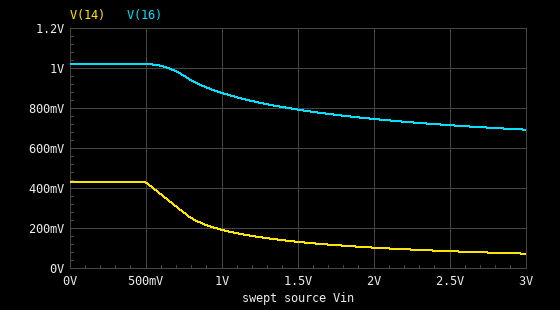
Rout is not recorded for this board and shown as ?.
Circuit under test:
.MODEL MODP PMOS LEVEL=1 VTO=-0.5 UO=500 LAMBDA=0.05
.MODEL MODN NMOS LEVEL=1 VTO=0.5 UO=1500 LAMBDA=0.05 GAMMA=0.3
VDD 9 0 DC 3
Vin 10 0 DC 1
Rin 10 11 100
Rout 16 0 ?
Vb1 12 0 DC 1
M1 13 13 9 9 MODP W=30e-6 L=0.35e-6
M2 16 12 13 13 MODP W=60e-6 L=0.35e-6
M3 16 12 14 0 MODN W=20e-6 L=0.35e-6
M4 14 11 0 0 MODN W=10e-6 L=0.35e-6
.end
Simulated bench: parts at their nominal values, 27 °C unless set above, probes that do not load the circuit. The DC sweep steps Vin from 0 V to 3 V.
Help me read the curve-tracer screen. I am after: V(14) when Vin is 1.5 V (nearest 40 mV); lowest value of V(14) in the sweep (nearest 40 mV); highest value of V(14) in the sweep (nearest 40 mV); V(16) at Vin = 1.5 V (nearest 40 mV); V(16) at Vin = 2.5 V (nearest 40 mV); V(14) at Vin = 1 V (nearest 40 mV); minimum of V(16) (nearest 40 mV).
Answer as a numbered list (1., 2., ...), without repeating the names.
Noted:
1. 120 mV
2. 80 mV
3. 440 mV
4. 800 mV
5. 720 mV
6. 200 mV
7. 680 mV
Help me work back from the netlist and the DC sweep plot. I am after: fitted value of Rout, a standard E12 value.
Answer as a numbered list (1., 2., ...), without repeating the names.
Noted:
1. 3.3 kΩ
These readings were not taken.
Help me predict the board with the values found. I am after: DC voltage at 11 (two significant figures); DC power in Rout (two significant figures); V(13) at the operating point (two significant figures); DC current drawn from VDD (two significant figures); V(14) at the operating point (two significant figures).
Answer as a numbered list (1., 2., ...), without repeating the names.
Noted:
1. 1.0 V
2. 230 µW
3. 1.9 V
4. 310 µA
5. 190 mV
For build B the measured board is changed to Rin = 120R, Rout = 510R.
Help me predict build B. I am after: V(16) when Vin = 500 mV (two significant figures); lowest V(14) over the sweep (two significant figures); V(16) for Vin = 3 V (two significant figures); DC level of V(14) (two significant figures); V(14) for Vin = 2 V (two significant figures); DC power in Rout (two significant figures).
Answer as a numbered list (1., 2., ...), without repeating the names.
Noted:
1. 160 mV
2. 34 mV
3. 140 mV
4. 91 mV
5. 49 mV
6. 43 µW
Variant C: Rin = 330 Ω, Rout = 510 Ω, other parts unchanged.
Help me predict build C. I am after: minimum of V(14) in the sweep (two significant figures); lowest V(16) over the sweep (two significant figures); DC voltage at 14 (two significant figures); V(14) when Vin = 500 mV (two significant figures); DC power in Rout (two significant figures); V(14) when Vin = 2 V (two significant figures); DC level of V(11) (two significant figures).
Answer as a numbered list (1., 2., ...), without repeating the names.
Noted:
1. 34 mV
2. 140 mV
3. 91 mV
4. 160 mV
5. 43 µW
6. 49 mV
7. 1.0 V
